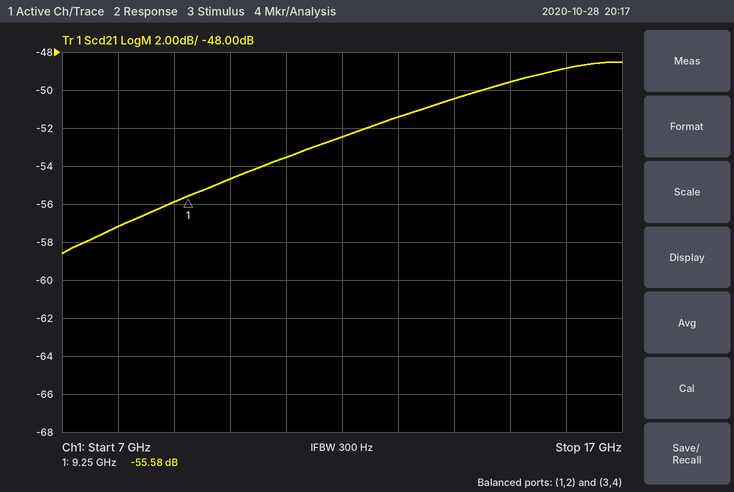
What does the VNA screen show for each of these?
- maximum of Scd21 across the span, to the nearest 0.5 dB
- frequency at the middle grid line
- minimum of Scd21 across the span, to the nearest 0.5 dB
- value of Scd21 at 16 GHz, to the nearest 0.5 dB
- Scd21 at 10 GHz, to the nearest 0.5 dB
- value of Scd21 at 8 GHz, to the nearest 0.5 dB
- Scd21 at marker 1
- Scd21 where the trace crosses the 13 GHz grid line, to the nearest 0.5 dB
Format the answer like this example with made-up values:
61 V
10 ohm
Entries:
-48.5 dB
12 GHz
-58.5 dB
-49.0 dB
-54.5 dB
-57.0 dB
-55.58 dB
-51.5 dB
